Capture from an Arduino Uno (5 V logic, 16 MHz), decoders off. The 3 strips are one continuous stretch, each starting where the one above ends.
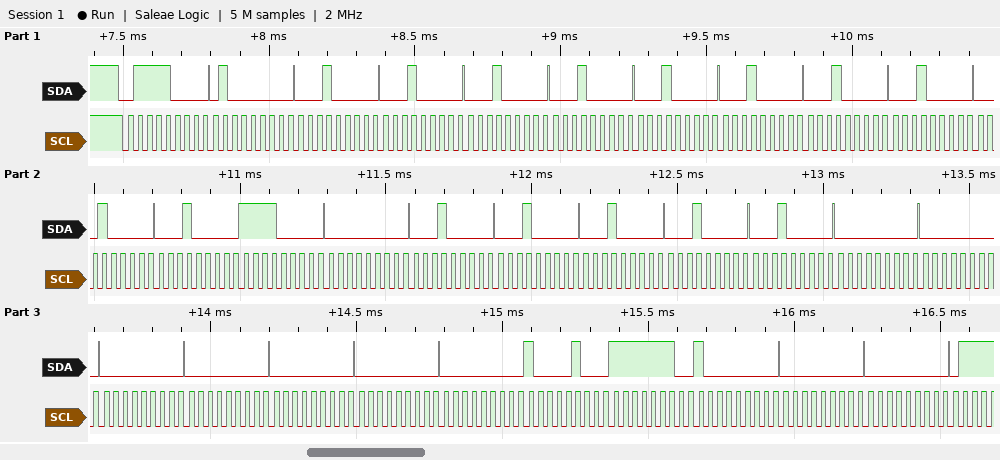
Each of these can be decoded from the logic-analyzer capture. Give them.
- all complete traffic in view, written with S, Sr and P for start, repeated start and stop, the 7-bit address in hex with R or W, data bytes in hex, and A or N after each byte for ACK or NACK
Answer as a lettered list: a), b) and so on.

a) S 3CW A 40 A 10 A 10 A 10 A 10 A 10 A 10 A 10 A 10 A 10 A 10 A F0 A 00 A 10 A 10 A 10 A 10 A 10 A 00 A 00 A 00 A 00 A 00 A 00 A 00 A 84 A FE A 80 A 00 A 00 A
